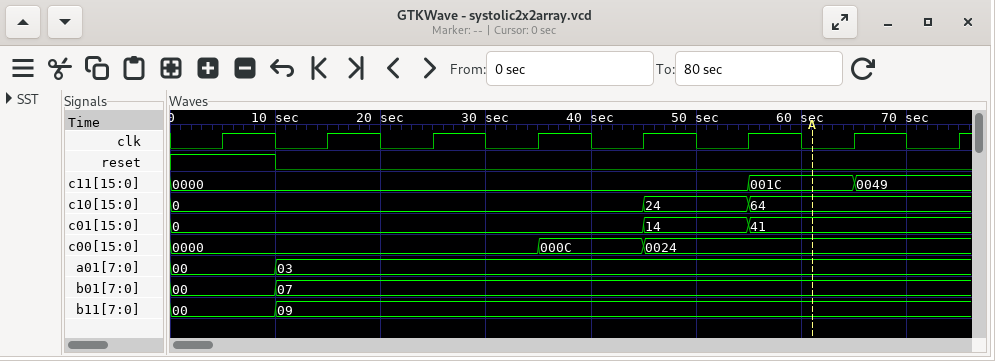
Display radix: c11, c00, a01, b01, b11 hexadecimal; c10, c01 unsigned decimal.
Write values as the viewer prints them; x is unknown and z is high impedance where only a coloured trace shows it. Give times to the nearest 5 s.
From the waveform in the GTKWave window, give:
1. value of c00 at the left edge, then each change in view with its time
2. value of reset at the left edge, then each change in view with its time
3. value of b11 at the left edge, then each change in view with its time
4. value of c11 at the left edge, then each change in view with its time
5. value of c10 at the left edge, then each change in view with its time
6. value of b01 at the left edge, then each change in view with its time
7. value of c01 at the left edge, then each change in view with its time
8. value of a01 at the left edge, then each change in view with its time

0000, 000C at 35 s, 0024 at 45 s
1, 0 at 10 s
00, 09 at 10 s
0000, 001C at 55 s, 0049 at 65 s
0, 24 at 45 s, 64 at 55 s
00, 07 at 10 s
0, 14 at 45 s, 41 at 55 s
00, 03 at 10 s
